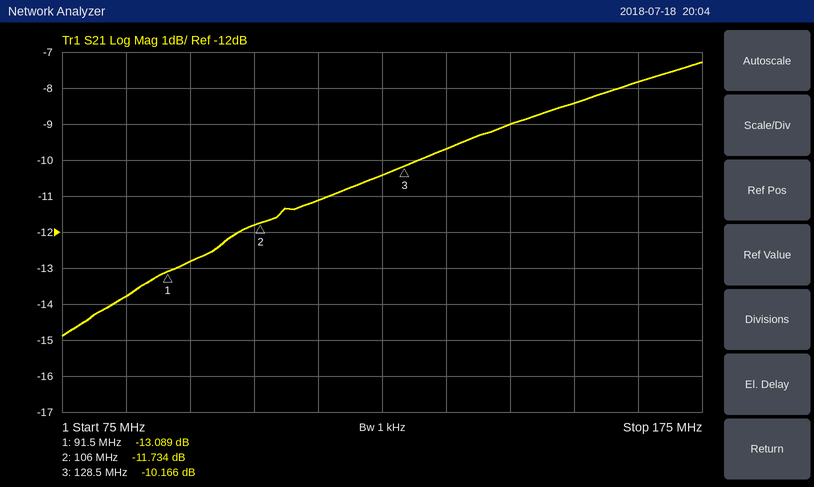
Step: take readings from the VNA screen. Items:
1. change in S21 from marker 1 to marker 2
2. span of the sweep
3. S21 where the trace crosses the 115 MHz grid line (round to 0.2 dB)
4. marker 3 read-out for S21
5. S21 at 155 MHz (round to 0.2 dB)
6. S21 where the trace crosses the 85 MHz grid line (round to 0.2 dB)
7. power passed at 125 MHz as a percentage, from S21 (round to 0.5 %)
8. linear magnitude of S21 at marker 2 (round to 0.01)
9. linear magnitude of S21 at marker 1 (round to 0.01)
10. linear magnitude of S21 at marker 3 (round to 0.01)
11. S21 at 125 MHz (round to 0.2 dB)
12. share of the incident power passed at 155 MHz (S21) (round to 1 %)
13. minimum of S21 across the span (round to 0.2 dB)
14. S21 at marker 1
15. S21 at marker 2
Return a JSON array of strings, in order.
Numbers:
["1.355 dB", "100 MHz", "-11.2 dB", "-10.166 dB", "-8.4 dB", "-13.8 dB", "9.0 %", "0.26", "0.22", "0.31", "-10.4 dB", "14 %", "-14.8 dB", "-13.089 dB", "-11.734 dB"]
